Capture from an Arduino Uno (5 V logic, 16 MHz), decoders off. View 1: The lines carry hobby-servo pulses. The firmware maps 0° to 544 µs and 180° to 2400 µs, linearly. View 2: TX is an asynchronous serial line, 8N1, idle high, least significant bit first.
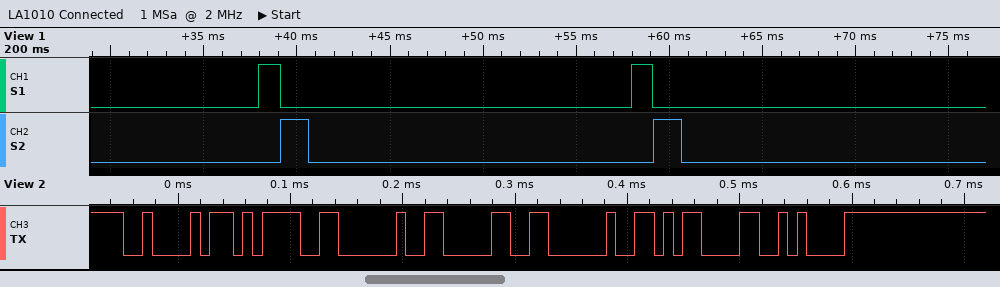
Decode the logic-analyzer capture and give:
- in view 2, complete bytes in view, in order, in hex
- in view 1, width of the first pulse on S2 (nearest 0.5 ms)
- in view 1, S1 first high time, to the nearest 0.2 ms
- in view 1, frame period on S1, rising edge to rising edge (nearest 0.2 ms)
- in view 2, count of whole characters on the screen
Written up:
42 3D 20 30 20 0D 0A
1.5 ms
1.2 ms
20.0 ms
7
